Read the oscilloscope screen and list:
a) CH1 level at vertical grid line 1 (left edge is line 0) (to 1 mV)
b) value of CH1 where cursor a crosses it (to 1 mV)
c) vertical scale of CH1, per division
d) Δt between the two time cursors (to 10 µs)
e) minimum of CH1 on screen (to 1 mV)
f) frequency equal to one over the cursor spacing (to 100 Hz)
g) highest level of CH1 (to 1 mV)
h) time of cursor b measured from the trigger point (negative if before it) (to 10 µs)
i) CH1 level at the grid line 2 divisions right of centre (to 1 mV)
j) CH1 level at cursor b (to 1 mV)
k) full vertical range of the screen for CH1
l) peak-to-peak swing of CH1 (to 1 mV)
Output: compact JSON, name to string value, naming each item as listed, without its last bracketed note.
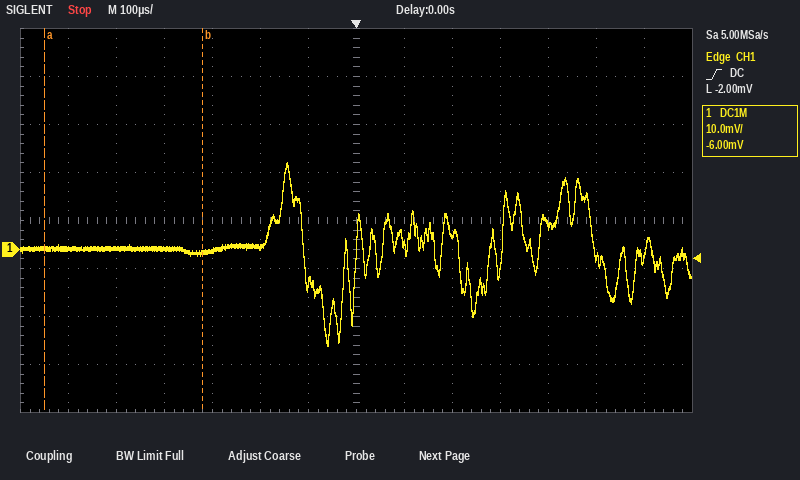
{"CH1 level at vertical grid line 1 (left edge is line 0)": "0 mV", "value of CH1 where cursor a crosses it": "0 mV", "vertical scale of CH1, per division": "10 mV", "Δt between the two time cursors": "330 µs", "minimum of CH1 on screen": "-20 mV", "frequency equal to one over the cursor spacing": "3.0 kHz", "highest level of CH1": "18 mV", "time of cursor b measured from the trigger point (negative if before it)": "-320 µs", "CH1 level at the grid line 2 divisions right of centre": "3 mV", "CH1 level at cursor b": "-1 mV", "full vertical range of the screen for CH1": "80 mV", "peak-to-peak swing of CH1": "38 mV"}
